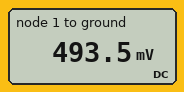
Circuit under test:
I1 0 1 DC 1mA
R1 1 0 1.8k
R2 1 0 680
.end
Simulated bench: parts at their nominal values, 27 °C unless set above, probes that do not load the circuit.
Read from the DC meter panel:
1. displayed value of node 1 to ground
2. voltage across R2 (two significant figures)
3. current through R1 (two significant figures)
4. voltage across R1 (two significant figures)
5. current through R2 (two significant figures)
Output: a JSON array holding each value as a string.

["493.5 mV", "490 mV", "270 µA", "490 mV", "730 µA"]
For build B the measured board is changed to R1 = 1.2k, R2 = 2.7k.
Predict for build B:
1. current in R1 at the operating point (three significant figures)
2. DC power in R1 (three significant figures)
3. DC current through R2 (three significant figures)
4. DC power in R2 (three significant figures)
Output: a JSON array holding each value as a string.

["692 µA", "575 µW", "308 µA", "256 µW"]
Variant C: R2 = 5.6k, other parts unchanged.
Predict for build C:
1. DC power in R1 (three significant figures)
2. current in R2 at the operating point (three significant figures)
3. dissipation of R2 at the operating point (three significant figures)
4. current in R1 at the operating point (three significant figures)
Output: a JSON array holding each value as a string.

["1.03 mW", "243 µA", "331 µW", "757 µA"]
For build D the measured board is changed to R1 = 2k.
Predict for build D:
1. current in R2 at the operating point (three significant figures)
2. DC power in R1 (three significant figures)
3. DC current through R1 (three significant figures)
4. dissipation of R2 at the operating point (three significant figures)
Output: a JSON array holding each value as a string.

["746 µA", "129 µW", "254 µA", "379 µW"]
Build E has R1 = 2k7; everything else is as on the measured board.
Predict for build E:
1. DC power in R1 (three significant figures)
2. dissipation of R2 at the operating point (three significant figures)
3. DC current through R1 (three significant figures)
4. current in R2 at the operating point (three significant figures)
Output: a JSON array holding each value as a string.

["109 µW", "434 µW", "201 µA", "799 µA"]
